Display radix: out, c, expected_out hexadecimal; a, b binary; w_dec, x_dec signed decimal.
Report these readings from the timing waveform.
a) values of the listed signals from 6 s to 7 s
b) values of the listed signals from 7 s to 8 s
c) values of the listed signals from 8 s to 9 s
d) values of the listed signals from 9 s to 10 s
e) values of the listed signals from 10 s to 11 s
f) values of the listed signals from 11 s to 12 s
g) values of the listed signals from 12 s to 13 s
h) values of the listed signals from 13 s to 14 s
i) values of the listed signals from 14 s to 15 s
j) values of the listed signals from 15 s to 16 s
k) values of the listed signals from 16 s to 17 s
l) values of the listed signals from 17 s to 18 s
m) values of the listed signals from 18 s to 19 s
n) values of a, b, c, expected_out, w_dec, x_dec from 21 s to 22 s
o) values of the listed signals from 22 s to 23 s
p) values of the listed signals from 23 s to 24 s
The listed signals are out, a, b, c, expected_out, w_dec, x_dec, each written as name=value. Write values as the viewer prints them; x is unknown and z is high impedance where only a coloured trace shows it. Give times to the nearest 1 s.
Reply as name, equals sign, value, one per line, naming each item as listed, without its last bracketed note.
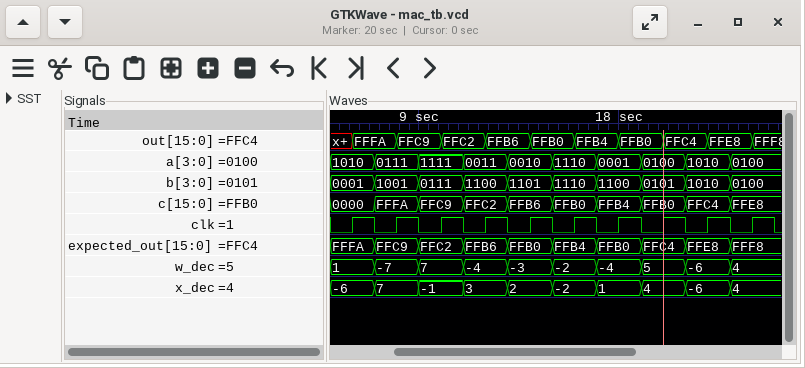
values of the listed signals from 6 s to 7 s = out=FFFA, a=1010, b=0001, c=0000, expected_out=FFFA, w_dec=1, x_dec=-6
values of the listed signals from 7 s to 8 s = out=FFFA, a=0111, b=1001, c=FFFA, expected_out=FFC9, w_dec=-7, x_dec=7
values of the listed signals from 8 s to 9 s = out=FFC9, a=0111, b=1001, c=FFFA, expected_out=FFC9, w_dec=-7, x_dec=7
values of the listed signals from 9 s to 10 s = out=FFC9, a=1111, b=0111, c=FFC9, expected_out=FFC2, w_dec=7, x_dec=-1
values of the listed signals from 10 s to 11 s = out=FFC2, a=1111, b=0111, c=FFC9, expected_out=FFC2, w_dec=7, x_dec=-1
values of the listed signals from 11 s to 12 s = out=FFC2, a=0011, b=1100, c=FFC2, expected_out=FFB6, w_dec=-4, x_dec=3
values of the listed signals from 12 s to 13 s = out=FFB6, a=0011, b=1100, c=FFC2, expected_out=FFB6, w_dec=-4, x_dec=3
values of the listed signals from 13 s to 14 s = out=FFB6, a=0010, b=1101, c=FFB6, expected_out=FFB0, w_dec=-3, x_dec=2
values of the listed signals from 14 s to 15 s = out=FFB0, a=0010, b=1101, c=FFB6, expected_out=FFB0, w_dec=-3, x_dec=2
values of the listed signals from 15 s to 16 s = out=FFB0, a=1110, b=1110, c=FFB0, expected_out=FFB4, w_dec=-2, x_dec=-2
values of the listed signals from 16 s to 17 s = out=FFB4, a=1110, b=1110, c=FFB0, expected_out=FFB4, w_dec=-2, x_dec=-2
values of the listed signals from 17 s to 18 s = out=FFB4, a=0001, b=1100, c=FFB4, expected_out=FFB0, w_dec=-4, x_dec=1
values of the listed signals from 18 s to 19 s = out=FFB0, a=0001, b=1100, c=FFB4, expected_out=FFB0, w_dec=-4, x_dec=1
values of a, b, c, expected_out, w_dec, x_dec from 21 s to 22 s = a=1010, b=1010, c=FFC4, expected_out=FFE8, w_dec=-6, x_dec=-6
values of the listed signals from 22 s to 23 s = out=FFE8, a=1010, b=1010, c=FFC4, expected_out=FFE8, w_dec=-6, x_dec=-6
values of the listed signals from 23 s to 24 s = out=FFE8, a=0100, b=0100, c=FFE8, expected_out=FFF8, w_dec=4, x_dec=4
